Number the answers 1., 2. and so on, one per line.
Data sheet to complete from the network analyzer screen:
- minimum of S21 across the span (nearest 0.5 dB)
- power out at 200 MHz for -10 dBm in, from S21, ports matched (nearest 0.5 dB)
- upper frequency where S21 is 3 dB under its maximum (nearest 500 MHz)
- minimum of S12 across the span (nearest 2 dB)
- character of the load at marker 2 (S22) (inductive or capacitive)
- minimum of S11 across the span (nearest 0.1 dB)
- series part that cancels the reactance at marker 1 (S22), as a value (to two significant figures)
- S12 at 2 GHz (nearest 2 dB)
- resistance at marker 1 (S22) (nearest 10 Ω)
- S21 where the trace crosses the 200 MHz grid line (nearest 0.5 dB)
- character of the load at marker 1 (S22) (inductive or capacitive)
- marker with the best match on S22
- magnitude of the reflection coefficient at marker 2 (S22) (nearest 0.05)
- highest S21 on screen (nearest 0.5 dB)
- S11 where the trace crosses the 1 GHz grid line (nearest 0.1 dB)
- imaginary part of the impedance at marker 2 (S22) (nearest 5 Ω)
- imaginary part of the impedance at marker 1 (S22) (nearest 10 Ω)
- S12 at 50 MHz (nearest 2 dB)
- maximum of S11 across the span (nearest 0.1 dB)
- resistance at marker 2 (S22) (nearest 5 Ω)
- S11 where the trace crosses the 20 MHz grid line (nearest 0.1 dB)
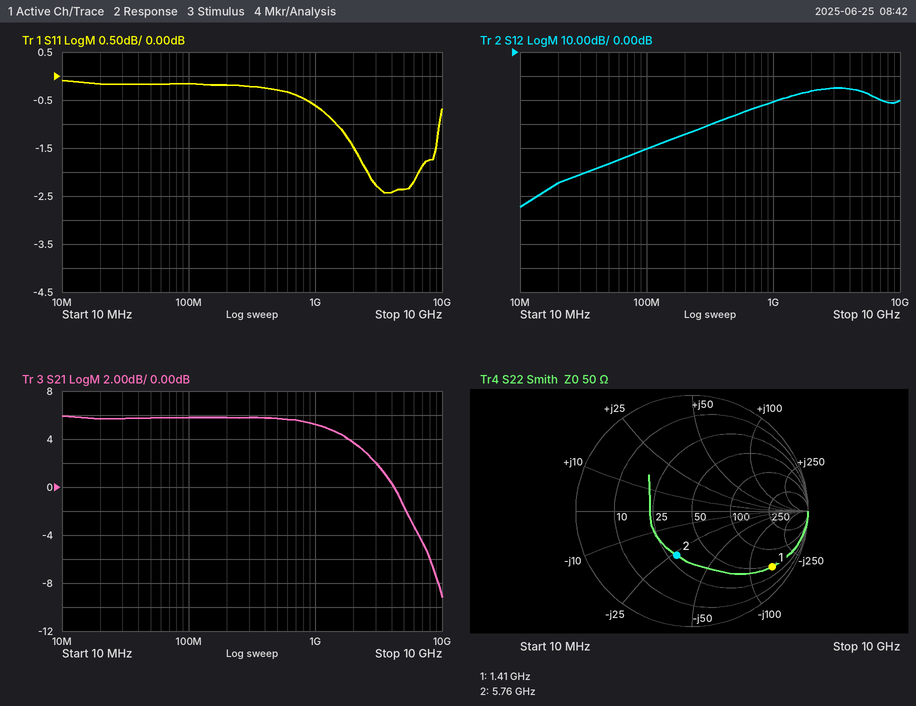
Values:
1. -9.0 dB
2. -4.0 dBm
3. 2.5 GHz
4. -64 dB
5. capacitive
6. -2.4 dB
7. 17 nH
8. -16 dB
9. 40 Ω
10. 6.0 dB
11. capacitive
12. marker 2
13. 0.40
14. 6.0 dB
15. -0.6 dB
16. -25 Ω
17. -150 Ω
18. -46 dB
19. -0.1 dB
20. 30 Ω
21. -0.2 dB
